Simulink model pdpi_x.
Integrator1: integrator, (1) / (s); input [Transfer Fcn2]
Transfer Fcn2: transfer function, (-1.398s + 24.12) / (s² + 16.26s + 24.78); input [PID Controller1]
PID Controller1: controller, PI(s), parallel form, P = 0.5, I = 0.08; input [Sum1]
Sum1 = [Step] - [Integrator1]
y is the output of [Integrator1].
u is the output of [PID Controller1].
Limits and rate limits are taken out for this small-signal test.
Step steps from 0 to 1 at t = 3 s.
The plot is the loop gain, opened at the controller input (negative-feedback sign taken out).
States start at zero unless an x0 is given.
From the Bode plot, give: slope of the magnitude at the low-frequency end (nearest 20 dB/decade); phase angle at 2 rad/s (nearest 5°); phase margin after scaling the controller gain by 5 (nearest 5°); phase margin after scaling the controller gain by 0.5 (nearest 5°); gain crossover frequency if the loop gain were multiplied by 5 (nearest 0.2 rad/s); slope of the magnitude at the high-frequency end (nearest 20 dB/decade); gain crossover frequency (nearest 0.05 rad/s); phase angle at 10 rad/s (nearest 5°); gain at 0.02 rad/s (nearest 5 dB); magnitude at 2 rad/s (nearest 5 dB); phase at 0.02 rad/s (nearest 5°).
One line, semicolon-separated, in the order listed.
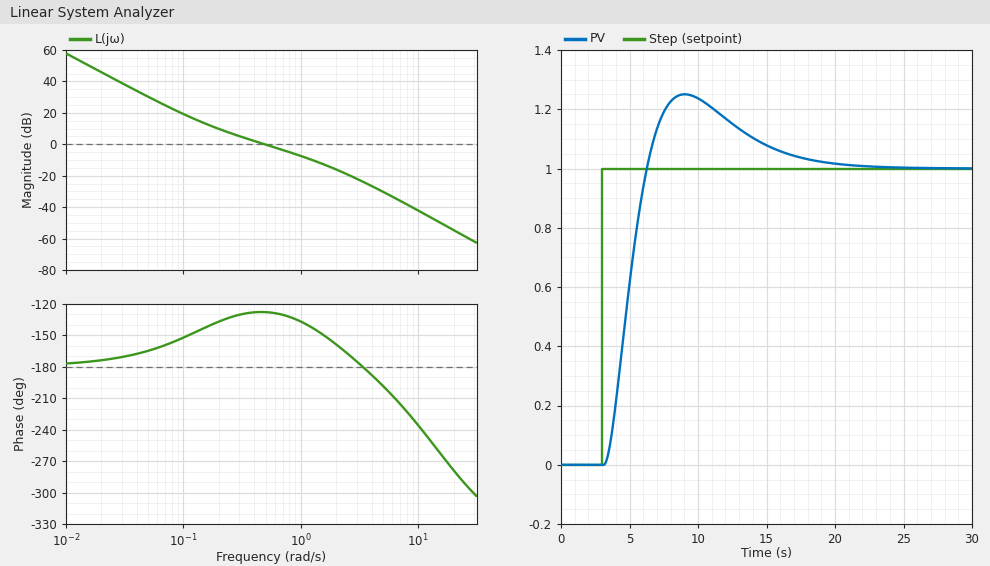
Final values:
-40 dB/decade; -160°; 25°; 50°; 1.8 rad/s; -40 dB/decade; 0.50 rad/s; -235°; 45 dB; -15 dB; -175°
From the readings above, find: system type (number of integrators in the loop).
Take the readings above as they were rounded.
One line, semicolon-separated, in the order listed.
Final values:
2
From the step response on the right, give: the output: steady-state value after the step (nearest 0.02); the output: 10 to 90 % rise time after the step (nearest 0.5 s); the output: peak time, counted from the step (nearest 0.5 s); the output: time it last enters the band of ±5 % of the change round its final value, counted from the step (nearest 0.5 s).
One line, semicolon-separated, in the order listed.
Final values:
1.00; 2.0 s; 6.0 s; 13.5 s
